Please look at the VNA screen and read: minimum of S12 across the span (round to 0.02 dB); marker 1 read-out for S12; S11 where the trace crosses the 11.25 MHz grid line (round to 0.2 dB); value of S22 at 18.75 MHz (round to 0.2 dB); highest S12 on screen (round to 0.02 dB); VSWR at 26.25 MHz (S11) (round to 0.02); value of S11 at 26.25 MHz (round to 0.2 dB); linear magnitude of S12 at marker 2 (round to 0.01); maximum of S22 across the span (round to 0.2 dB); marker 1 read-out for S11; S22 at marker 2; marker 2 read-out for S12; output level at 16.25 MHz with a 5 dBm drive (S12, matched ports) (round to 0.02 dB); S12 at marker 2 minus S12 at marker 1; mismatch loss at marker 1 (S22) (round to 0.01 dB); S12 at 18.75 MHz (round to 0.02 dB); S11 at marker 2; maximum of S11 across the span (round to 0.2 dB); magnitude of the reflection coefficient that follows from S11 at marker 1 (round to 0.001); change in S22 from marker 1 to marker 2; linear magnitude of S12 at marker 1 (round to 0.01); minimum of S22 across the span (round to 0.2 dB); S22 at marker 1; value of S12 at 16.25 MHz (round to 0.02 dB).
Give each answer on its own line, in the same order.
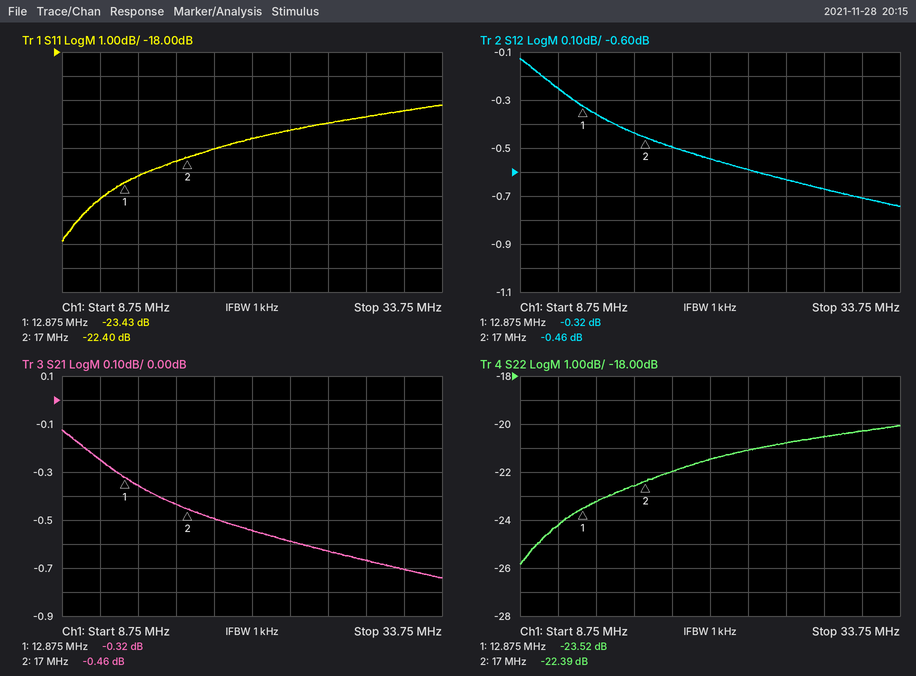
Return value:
-0.74 dB
-0.32 dB
-24.2 dB
-22.0 dB
-0.12 dB
1.20
-21.0 dB
0.95
-20.0 dB
-23.43 dB
-22.39 dB
-0.46 dB
4.56 dBm
-0.14 dB
0.02 dB
-0.50 dB
-22.40 dB
-20.2 dB
0.067
1.13 dB
0.96
-25.8 dB
-23.52 dB
-0.44 dB
